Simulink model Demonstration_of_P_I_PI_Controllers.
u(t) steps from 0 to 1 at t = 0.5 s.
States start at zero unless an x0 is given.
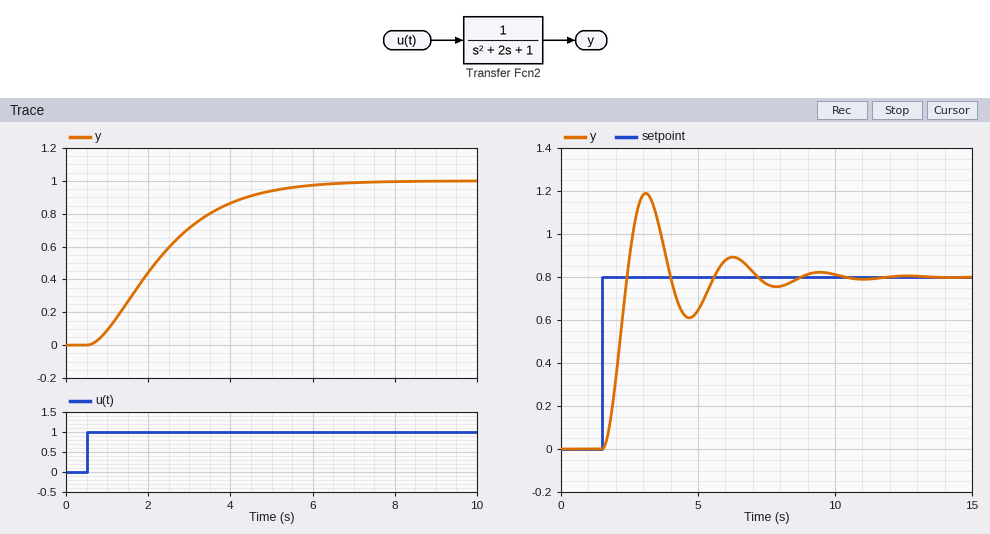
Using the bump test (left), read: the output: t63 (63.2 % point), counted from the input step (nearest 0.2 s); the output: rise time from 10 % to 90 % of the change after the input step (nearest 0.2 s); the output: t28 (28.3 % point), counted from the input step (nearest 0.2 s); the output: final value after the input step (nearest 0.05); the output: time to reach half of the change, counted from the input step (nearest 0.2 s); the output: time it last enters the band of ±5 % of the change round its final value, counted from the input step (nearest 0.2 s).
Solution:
2.2 s
3.4 s
1.0 s
1.00
1.6 s
4.8 s
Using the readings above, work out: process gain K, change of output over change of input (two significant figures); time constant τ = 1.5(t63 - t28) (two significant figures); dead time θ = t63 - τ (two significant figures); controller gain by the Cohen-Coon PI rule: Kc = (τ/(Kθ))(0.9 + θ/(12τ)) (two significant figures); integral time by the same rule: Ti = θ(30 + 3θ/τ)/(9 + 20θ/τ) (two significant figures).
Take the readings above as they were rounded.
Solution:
1.0
1.8 s
0.40 s
4.1
0.91 s
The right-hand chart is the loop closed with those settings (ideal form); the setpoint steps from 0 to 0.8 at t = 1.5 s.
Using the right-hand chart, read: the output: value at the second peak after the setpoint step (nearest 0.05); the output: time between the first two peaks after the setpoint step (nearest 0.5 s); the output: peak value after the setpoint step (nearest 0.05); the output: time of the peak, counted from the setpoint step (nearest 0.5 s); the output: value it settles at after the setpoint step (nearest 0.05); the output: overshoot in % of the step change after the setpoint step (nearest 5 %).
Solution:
0.90
3.0 s
1.20
1.5 s
0.80
50 %
